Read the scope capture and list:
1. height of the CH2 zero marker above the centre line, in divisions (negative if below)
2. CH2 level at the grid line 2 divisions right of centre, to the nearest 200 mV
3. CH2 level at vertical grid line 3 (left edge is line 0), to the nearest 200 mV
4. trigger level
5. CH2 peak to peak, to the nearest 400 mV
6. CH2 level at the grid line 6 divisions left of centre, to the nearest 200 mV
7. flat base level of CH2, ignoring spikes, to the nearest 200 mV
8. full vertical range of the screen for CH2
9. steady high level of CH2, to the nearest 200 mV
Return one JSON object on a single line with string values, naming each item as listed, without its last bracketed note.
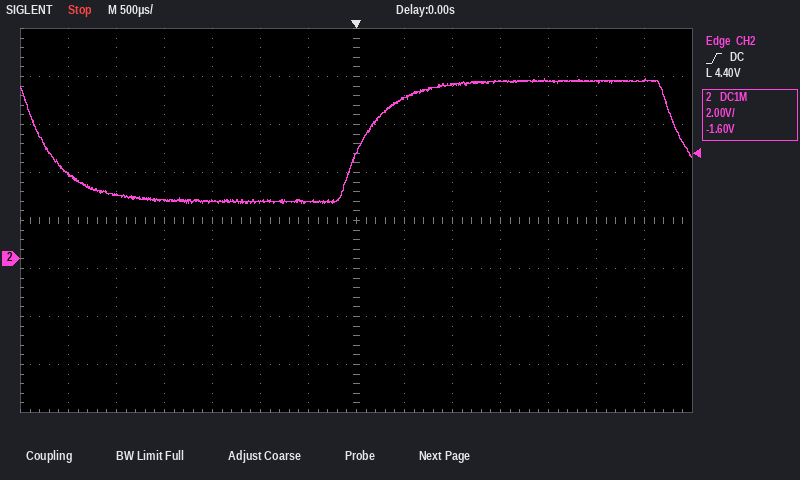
{"height of the CH2 zero marker above the centre line, in divisions": "-0.8 div", "CH2 level at the grid line 2 divisions right of centre, to the nearest 200 mV": "7.2 V", "CH2 level at vertical grid line 3 (left edge is line 0), to the nearest 200 mV": "2.4 V", "trigger level": "4.40 V", "CH2 peak to peak, to the nearest 400 mV": "5.2 V", "CH2 level at the grid line 6 divisions left of centre, to the nearest 200 mV": "3.6 V", "flat base level of CH2, ignoring spikes, to the nearest 200 mV": "2.4 V", "full vertical range of the screen for CH2": "16 V", "steady high level of CH2, to the nearest 200 mV": "7.4 V"}
